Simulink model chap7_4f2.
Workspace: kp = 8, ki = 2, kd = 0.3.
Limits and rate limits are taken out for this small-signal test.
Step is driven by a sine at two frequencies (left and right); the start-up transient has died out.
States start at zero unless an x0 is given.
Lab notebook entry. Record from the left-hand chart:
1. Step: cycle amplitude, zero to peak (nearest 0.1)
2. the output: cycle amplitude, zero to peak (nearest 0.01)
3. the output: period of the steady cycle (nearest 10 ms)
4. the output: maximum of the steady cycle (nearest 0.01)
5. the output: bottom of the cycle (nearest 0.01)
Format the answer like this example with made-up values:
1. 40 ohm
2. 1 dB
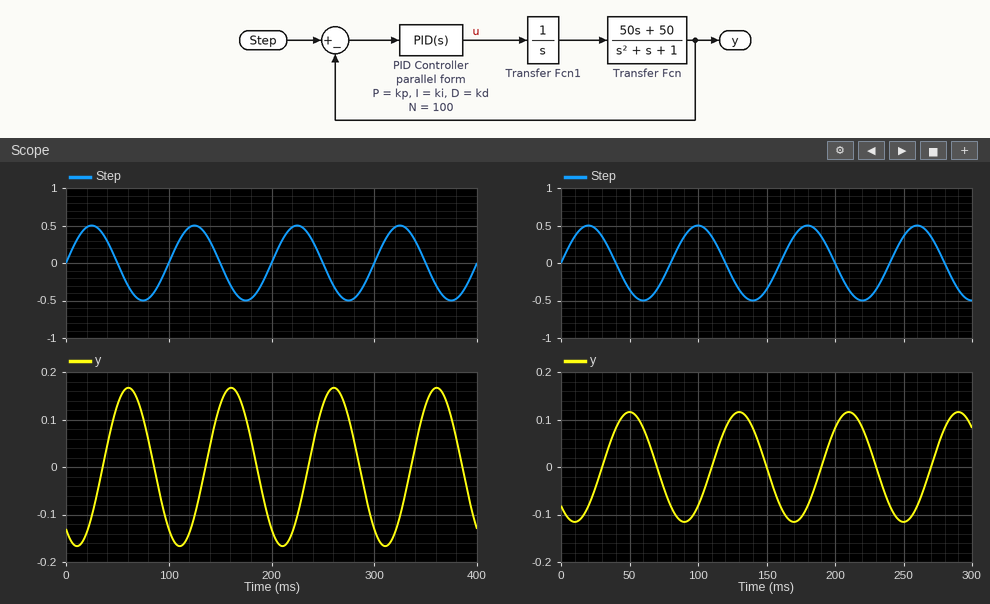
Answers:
1. 0.5
2. 0.17
3. 100 ms
4. 0.17
5. -0.17
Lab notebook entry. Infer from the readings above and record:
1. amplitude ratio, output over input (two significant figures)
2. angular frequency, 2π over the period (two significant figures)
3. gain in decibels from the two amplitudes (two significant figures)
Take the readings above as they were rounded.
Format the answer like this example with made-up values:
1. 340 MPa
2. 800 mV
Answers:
1. 0.34
2. 0.063 rad/ms
3. -9.4 dB
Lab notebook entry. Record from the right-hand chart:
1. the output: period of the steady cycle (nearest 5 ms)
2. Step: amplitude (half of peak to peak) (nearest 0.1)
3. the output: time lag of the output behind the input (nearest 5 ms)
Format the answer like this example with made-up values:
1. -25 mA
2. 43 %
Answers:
1. 80 ms
2. 0.5
3. 30 ms
